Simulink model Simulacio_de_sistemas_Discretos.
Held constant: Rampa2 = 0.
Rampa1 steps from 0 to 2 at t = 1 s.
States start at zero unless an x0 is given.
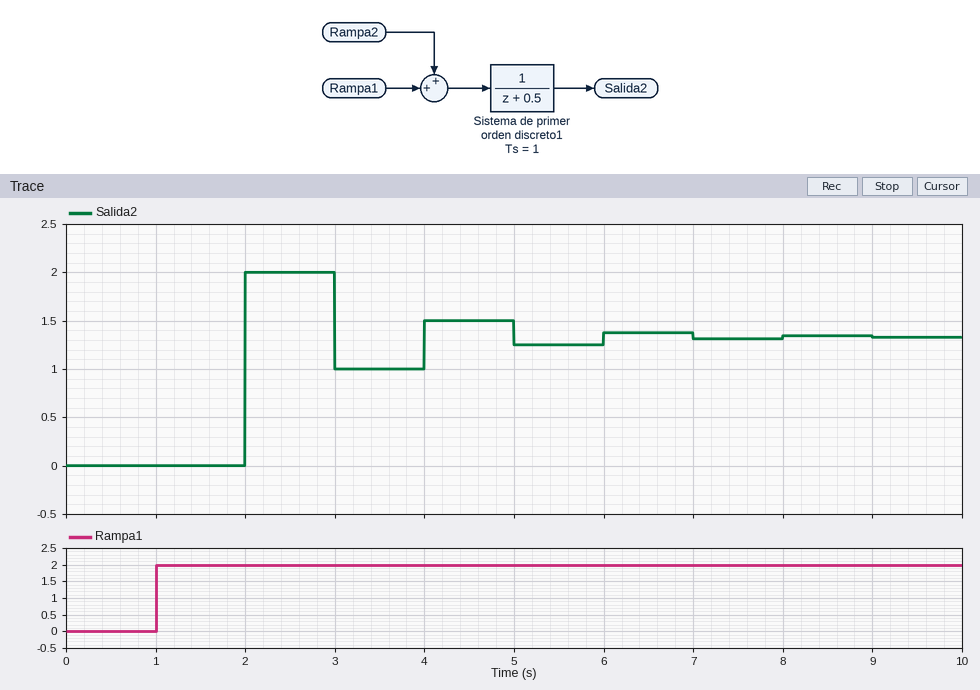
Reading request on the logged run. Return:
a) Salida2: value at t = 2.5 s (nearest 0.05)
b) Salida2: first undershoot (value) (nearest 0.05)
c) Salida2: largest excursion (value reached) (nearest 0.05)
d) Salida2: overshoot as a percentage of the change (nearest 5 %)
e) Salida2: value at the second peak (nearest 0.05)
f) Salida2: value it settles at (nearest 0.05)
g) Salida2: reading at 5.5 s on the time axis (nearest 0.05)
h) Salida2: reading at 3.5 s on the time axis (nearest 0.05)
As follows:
2.00
1.00
2.00
50 %
1.50
1.35
1.25
1.00
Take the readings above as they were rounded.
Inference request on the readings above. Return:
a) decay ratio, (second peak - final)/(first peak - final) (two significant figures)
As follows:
0.23
